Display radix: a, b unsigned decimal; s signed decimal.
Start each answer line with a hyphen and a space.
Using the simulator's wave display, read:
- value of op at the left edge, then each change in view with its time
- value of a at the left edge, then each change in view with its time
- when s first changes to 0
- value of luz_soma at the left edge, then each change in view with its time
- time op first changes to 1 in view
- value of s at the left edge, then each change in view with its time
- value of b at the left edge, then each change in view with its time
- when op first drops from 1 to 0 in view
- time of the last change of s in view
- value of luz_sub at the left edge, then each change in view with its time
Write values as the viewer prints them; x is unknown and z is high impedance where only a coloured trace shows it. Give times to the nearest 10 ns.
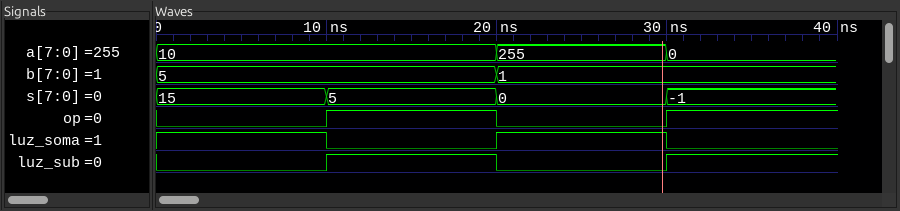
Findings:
- 0, 1 at 10 ns, 0 at 20 ns, 1 at 30 ns
- 10, 255 at 20 ns, 0 at 30 ns
- 20 ns
- 1, 0 at 10 ns, 1 at 20 ns, 0 at 30 ns
- 10 ns
- 15, 5 at 10 ns, 0 at 20 ns, -1 at 30 ns
- 5, 1 at 20 ns
- 20 ns
- 30 ns
- 0, 1 at 10 ns, 0 at 20 ns, 1 at 30 ns
